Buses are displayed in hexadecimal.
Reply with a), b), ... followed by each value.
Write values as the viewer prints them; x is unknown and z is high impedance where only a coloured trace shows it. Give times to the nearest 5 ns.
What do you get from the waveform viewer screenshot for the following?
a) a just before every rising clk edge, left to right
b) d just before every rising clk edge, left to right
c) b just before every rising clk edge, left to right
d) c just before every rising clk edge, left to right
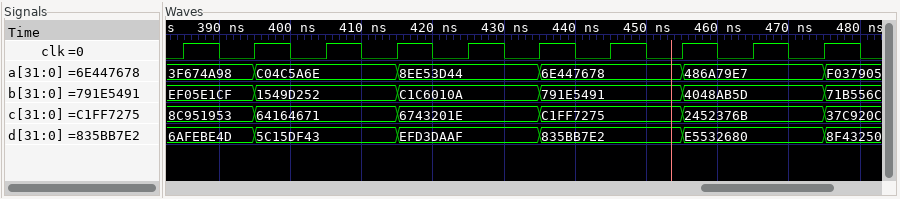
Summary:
a) 3F674A98, 3F674A98, C04C5A6E, C04C5A6E, 8EE53D44, 8EE53D44, 6E447678, 6E447678, 486A79E7, 486A79E7
b) 6AFEBE4D, 6AFEBE4D, 5C15DF43, 5C15DF43, EFD3DAAF, EFD3DAAF, 835BB7E2, 835BB7E2, E5532680, E5532680
c) EF05E1CF, EF05E1CF, 1549D252, 1549D252, C1C6010A, C1C6010A, 791E5491, 791E5491, 4048AB5D, 4048AB5D
d) 8C951953, 8C951953, 64164671, 64164671, 6743201E, 6743201E, C1FF7275, C1FF7275, 2452376B, 2452376B
